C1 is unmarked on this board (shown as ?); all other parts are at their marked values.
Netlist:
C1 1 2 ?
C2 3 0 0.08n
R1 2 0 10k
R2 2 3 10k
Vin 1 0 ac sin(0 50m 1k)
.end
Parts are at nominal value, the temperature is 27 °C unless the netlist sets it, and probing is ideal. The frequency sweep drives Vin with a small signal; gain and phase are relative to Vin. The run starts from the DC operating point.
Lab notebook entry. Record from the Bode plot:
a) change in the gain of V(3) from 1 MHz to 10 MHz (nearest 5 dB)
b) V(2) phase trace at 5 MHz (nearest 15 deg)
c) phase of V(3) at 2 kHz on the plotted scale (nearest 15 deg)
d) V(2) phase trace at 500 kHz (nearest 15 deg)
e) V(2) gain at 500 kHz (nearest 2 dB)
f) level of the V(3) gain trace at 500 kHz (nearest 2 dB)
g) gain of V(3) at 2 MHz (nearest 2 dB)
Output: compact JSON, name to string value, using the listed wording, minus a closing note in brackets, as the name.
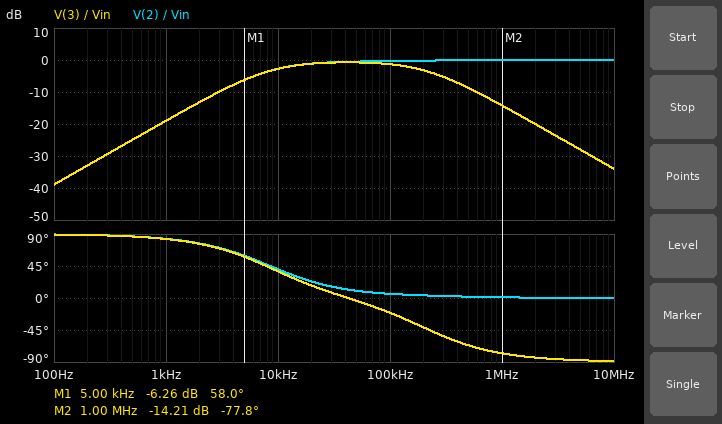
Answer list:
{"change in the gain of V(3) from 1 MHz to 10 MHz": "-20 dB", "V(2) phase trace at 5 MHz": "0 deg", "phase of V(3) at 2 kHz on the plotted scale": "75 deg", "V(2) phase trace at 500 kHz": "0 deg", "V(2) gain at 500 kHz": "0 dB", "level of the V(3) gain trace at 500 kHz": "-8 dB", "gain of V(3) at 2 MHz": "-20 dB"}
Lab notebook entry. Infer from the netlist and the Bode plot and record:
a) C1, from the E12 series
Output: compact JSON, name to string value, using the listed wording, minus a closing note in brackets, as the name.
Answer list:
{"C1, from the E12 series": "1.8 nF"}
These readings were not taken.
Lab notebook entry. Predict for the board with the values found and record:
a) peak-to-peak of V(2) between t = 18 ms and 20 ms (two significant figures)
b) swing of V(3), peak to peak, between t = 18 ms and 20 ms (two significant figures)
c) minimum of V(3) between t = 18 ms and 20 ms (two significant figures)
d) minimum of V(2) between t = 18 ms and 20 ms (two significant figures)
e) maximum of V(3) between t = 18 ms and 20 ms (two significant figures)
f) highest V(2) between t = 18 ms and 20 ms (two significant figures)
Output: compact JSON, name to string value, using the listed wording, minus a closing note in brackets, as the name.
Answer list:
{"peak-to-peak of V(2) between t = 18 ms and 20 ms": "11 mV", "swing of V(3), peak to peak, between t = 18 ms and 20 ms": "11 mV", "minimum of V(3) between t = 18 ms and 20 ms": "-5.6 mV", "minimum of V(2) between t = 18 ms and 20 ms": "-5.6 mV", "maximum of V(3) between t = 18 ms and 20 ms": "5.6 mV", "highest V(2) between t = 18 ms and 20 ms": "5.6 mV"}
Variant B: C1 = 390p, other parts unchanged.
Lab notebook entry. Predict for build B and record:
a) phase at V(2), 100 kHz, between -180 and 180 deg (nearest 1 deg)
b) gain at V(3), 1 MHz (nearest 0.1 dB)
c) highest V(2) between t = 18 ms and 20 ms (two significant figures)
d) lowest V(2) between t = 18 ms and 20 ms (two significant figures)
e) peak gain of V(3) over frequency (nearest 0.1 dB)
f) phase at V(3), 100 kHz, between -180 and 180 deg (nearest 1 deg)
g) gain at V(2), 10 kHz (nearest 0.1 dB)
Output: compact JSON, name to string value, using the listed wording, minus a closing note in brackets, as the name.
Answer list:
{"phase at V(2), 100 kHz, between -180 and 180 deg": "23 deg", "gain at V(3), 1 MHz": "-14.3 dB", "highest V(2) between t = 18 ms and 20 ms": "1.2 mV", "lowest V(2) between t = 18 ms and 20 ms": "-1.2 mV", "peak gain of V(3) over frequency": "-3.0 dB", "phase at V(3), 100 kHz, between -180 and 180 deg": "-4 deg", "gain at V(2), 10 kHz": "-12.6 dB"}
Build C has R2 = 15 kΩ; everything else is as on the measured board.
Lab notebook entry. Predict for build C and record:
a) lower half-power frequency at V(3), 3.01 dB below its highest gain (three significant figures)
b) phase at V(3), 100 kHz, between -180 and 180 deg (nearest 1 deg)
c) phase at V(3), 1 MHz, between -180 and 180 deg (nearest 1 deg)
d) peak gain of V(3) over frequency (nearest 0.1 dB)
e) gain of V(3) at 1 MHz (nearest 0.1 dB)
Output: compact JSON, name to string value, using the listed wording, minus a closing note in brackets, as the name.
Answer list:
{"lower half-power frequency at V(3), 3.01 dB below its highest gain": "7.57 kHz", "phase at V(3), 100 kHz, between -180 and 180 deg": "-31 deg", "phase at V(3), 1 MHz, between -180 and 180 deg": "-82 deg", "peak gain of V(3) over frequency": "-0.9 dB", "gain of V(3) at 1 MHz": "-17.6 dB"}
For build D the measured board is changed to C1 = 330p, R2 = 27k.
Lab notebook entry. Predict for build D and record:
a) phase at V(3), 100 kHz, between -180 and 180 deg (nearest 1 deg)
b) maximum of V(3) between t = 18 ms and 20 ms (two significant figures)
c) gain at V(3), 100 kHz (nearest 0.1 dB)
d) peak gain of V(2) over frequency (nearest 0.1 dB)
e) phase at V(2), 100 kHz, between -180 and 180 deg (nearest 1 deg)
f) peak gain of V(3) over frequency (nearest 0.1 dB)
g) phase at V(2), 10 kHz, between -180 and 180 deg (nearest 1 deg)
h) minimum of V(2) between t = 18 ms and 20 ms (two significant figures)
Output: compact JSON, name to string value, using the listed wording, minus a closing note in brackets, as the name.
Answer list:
{"phase at V(3), 100 kHz, between -180 and 180 deg": "-25 deg", "maximum of V(3) between t = 18 ms and 20 ms": "1.0 mV", "gain at V(3), 100 kHz": "-6.4 dB", "peak gain of V(2) over frequency": "0 dB", "phase at V(2), 100 kHz, between -180 and 180 deg": "29 deg", "peak gain of V(3) over frequency": "-5.6 dB", "phase at V(2), 10 kHz, between -180 and 180 deg": "76 deg", "minimum of V(2) between t = 18 ms and 20 ms": "-1.0 mV"}
